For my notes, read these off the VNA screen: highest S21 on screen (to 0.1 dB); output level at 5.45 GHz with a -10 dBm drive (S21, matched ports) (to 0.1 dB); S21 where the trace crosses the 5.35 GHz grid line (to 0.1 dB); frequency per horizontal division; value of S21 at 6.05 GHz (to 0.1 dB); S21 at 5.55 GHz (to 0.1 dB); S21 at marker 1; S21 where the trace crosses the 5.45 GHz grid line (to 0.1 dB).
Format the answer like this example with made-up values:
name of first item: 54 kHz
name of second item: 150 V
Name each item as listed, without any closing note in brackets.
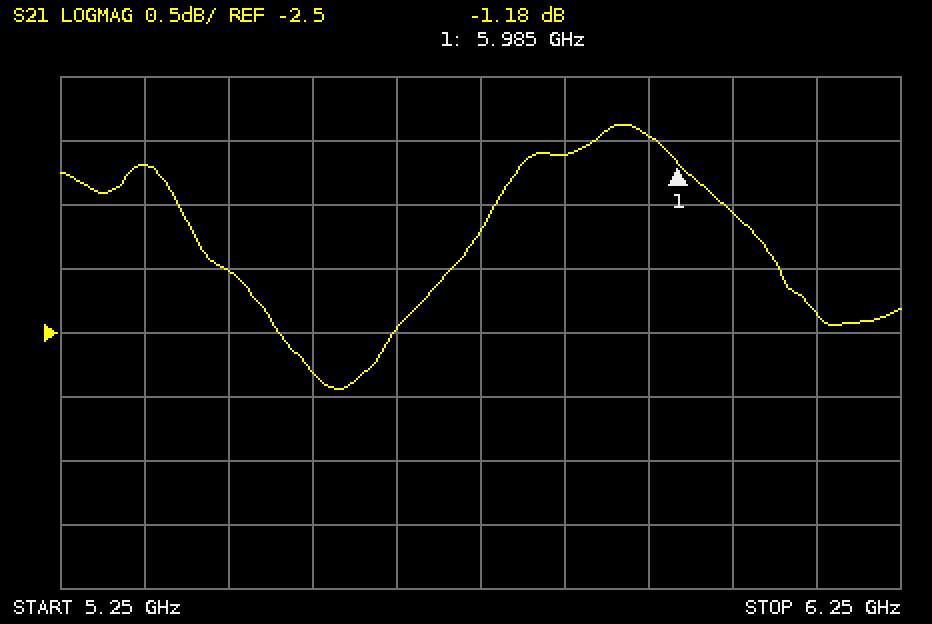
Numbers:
highest S21 on screen: -0.9 dB
output level at 5.45 GHz with a -10 dBm drive (S21, matched ports): -12.0 dBm
S21 where the trace crosses the 5.35 GHz grid line: -1.2 dB
frequency per horizontal division: 100 MHz
value of S21 at 6.05 GHz: -1.6 dB
S21 at 5.55 GHz: -2.8 dB
S21 at marker 1: -1.18 dB
S21 where the trace crosses the 5.45 GHz grid line: -2.0 dB
